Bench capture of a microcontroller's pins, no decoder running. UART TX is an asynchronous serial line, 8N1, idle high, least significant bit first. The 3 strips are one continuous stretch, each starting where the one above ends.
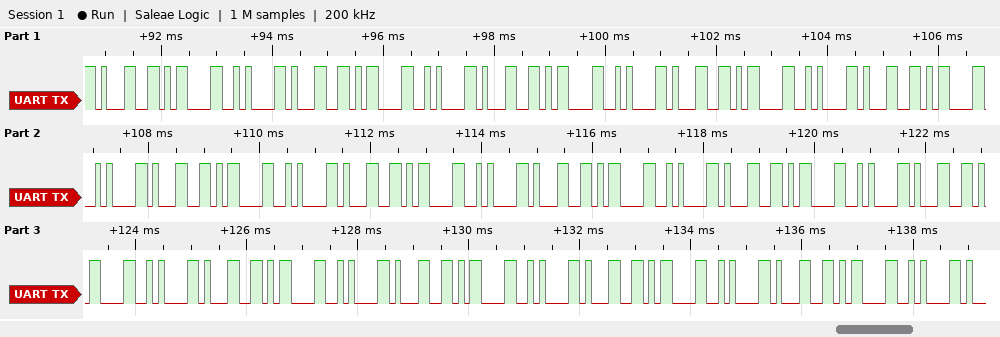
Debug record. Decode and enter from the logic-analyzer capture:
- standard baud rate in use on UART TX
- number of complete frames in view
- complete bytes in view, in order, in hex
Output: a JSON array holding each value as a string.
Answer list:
["9600 baud", "42", "31 0D 0A 31 0D 0A 31 0D 0A 31 0D 0A 31 0D 0A 31 0D 0A 31 0D 0A 31 0D 0A 31 0D 0A 31 0D 0A 31 0D 0A 31 0D 0A 31 0D 0A 31 0D 0A"]
